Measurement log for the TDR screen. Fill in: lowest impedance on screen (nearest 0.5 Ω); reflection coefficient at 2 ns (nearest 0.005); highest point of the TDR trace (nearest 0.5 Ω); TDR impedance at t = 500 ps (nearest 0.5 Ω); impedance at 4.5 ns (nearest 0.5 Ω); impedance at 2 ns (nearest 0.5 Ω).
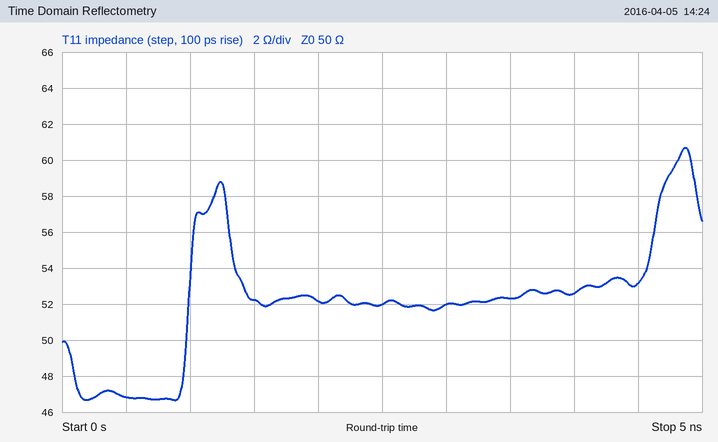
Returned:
46.5 Ω
+0.020
60.5 Ω
47.0 Ω
53.0 Ω
52.0 Ω
